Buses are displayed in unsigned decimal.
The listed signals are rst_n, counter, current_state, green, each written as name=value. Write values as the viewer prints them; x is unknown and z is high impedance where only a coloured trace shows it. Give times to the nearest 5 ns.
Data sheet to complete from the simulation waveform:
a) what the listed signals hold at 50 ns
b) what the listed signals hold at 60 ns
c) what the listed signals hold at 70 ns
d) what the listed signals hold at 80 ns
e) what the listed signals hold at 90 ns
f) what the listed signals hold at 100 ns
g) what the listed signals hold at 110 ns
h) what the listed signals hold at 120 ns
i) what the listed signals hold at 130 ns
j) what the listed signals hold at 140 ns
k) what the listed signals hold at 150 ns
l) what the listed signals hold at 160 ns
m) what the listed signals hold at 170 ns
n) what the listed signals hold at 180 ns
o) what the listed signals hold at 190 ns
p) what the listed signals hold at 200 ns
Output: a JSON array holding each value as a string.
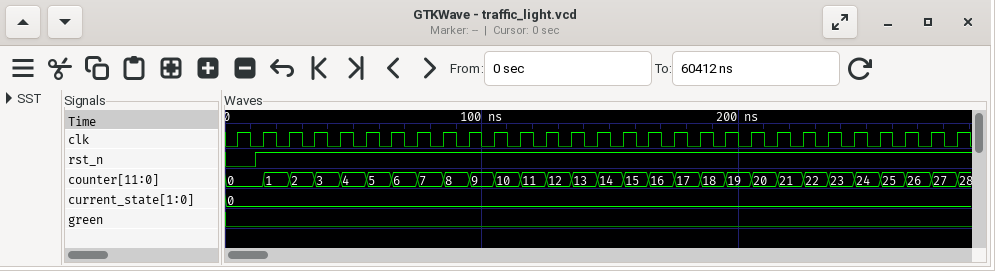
["rst_n=1, counter=4, current_state=0, green=0", "rst_n=1, counter=5, current_state=0, green=0", "rst_n=1, counter=6, current_state=0, green=0", "rst_n=1, counter=7, current_state=0, green=0", "rst_n=1, counter=8, current_state=0, green=0", "rst_n=1, counter=9, current_state=0, green=0", "rst_n=1, counter=10, current_state=0, green=0", "rst_n=1, counter=11, current_state=0, green=0", "rst_n=1, counter=12, current_state=0, green=0", "rst_n=1, counter=13, current_state=0, green=0", "rst_n=1, counter=14, current_state=0, green=0", "rst_n=1, counter=15, current_state=0, green=0", "rst_n=1, counter=16, current_state=0, green=0", "rst_n=1, counter=17, current_state=0, green=0", "rst_n=1, counter=18, current_state=0, green=0", "rst_n=1, counter=19, current_state=0, green=0"]
